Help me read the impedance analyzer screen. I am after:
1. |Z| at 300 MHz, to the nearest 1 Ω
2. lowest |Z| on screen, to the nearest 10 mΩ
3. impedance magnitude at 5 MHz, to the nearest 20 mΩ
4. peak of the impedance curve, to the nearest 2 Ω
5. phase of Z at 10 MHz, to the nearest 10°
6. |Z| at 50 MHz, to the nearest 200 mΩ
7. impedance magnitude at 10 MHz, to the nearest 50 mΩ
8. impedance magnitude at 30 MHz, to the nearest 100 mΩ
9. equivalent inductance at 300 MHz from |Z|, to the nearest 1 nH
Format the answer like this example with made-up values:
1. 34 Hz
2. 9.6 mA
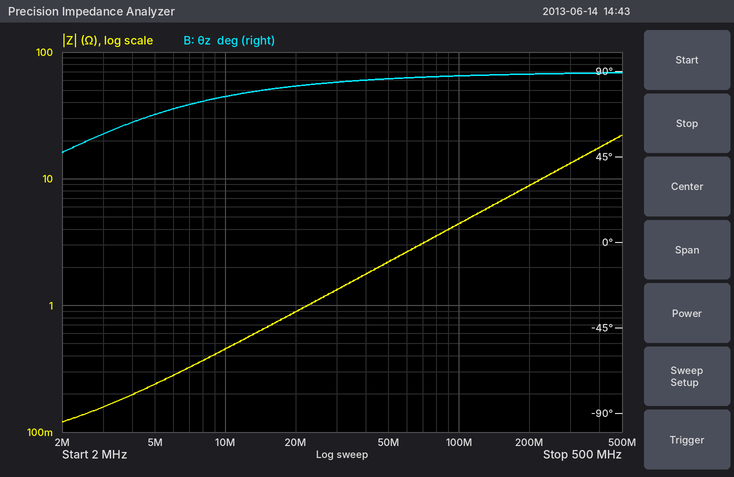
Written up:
1. 13 Ω
2. 120 mΩ
3. 240 mΩ
4. 22 Ω
5. 80°
6. 2.2 Ω
7. 450 mΩ
8. 1.3 Ω
9. 7 nH
